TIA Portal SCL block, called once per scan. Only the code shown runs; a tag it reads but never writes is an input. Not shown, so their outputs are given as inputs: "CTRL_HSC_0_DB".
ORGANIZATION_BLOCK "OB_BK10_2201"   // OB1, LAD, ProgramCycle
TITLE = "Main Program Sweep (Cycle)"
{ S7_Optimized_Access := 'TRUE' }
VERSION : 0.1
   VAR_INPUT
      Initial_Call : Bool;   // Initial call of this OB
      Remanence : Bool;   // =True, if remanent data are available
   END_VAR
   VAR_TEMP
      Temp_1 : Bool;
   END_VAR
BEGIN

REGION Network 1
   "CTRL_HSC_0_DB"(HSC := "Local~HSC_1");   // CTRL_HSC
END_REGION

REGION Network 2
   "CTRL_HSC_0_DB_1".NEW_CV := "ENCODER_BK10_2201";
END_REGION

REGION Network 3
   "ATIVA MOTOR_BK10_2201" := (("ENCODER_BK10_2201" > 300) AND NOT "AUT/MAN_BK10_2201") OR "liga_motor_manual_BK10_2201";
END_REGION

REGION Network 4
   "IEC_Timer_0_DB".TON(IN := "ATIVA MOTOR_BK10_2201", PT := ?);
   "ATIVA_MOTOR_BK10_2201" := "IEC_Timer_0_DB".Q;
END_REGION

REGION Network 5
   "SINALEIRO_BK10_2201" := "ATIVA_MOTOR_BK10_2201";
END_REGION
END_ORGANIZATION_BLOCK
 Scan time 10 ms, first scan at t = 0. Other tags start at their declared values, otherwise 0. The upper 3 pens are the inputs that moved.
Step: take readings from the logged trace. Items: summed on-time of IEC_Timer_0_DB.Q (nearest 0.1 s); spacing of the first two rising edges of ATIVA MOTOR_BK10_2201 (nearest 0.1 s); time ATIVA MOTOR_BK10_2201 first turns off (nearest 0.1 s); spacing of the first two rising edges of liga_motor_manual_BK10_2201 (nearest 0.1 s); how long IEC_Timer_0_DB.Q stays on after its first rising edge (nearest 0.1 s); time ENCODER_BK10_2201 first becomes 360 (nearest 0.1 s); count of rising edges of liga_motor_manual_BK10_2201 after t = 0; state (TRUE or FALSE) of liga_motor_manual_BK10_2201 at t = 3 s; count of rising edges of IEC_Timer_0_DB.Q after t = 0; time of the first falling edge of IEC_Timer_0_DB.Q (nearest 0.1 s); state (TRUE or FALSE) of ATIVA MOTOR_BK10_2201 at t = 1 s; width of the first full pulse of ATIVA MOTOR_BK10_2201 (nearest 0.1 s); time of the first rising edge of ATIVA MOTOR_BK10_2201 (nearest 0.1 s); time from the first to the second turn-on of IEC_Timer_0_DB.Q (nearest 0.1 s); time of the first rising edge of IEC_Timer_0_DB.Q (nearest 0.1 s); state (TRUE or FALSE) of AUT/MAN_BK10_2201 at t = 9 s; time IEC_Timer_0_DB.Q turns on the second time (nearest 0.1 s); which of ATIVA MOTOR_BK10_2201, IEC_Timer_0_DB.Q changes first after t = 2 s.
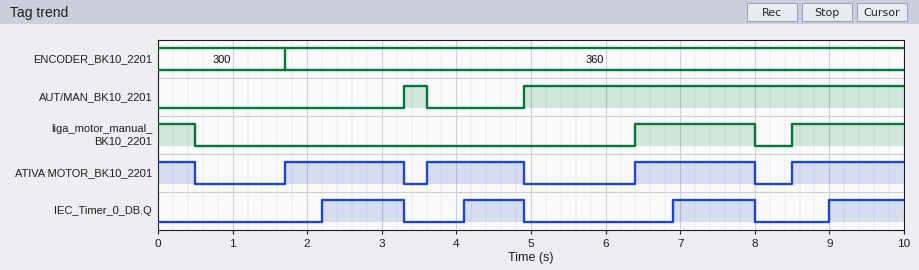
4.0 s
1.9 s
0.5 s
2.1 s
1.1 s
1.7 s
2
FALSE
4
3.3 s
FALSE
1.6 s
1.7 s
1.9 s
2.2 s
TRUE
4.1 s
IEC_Timer_0_DB.Q
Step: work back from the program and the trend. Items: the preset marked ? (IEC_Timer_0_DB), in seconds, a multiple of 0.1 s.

0.5 s
